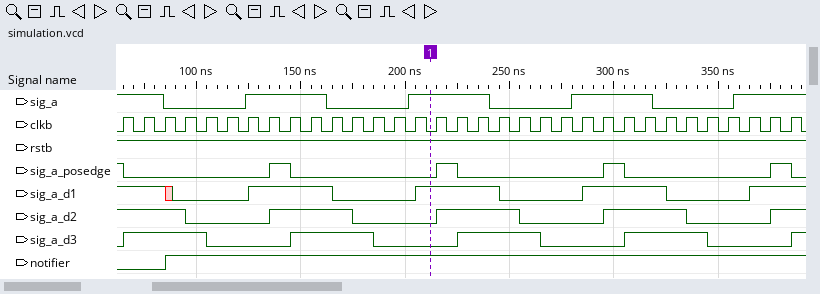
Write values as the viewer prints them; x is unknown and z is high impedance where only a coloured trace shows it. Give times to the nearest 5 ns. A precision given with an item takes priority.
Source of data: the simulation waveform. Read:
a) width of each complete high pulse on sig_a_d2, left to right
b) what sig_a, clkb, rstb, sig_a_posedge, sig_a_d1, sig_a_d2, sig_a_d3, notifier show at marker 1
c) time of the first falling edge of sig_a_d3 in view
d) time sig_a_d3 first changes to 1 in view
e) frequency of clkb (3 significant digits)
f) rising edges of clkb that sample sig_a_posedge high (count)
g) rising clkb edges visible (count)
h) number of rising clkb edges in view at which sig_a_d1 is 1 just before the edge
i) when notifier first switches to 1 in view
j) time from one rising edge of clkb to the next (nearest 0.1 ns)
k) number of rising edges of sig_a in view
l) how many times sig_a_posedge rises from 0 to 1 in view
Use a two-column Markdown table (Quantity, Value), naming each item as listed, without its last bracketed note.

| Quantity | Value |
|---|---|
| width of each complete high pulse on sig_a_d2, left to right | 40 ns, 40 ns, 40 ns |
| what sig_a, clkb, rstb, sig_a_posedge, sig_a_d1, sig_a_d2, sig_a_d3, notifier show at marker 1 | sig_a=1, clkb=0, rstb=1, sig_a_posedge=0, sig_a_d1=1, sig_a_d2=0, sig_a_d3=0, notifier=1 |
| time of the first falling edge of sig_a_d3 in view | 105 ns |
| time sig_a_d3 first changes to 1 in view | 65 ns |
| frequency of clkb | 100 MHz |
| rising edges of clkb that sample sig_a_posedge high | 5 |
| rising clkb edges visible | 33 |
| number of rising clkb edges in view at which sig_a_d1 is 1 just before the edge | 17 |
| when notifier first switches to 1 in view | 85 ns |
| time from one rising edge of clkb to the next | 10 ns |
| number of rising edges of sig_a in view | 4 |
| how many times sig_a_posedge rises from 0 to 1 in view | 4 |
